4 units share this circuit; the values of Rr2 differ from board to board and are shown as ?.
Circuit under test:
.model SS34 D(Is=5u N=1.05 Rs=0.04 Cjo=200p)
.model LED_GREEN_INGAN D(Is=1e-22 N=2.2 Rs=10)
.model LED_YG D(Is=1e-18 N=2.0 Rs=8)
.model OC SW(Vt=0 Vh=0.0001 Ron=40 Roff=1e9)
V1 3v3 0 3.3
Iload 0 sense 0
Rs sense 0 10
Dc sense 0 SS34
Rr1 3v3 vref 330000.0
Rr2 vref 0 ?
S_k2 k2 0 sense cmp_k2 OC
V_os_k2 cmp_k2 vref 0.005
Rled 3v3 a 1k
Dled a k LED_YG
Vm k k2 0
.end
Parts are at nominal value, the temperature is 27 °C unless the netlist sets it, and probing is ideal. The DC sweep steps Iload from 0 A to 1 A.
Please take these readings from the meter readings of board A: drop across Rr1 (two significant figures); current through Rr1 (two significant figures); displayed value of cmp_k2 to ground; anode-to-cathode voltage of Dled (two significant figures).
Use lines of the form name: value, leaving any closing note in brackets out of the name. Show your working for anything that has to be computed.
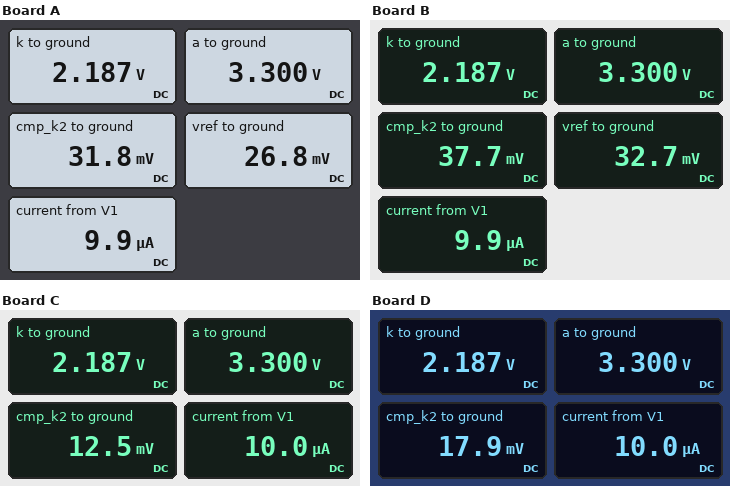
drop across Rr1: 3.3 V - 26.8 mV = 3.3 V
current through Rr1: (3.3 V - 26.8 mV) / 330 kΩ = 9.9 µA
displayed value of cmp_k2 to ground: 31.8 mV
anode-to-cathode voltage of Dled: 3.3 V - 2.187 V = 1.1 V
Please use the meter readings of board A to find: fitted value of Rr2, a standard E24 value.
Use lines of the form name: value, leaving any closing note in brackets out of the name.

fitted value of Rr2, a standard E24 value: 2.7 kΩ
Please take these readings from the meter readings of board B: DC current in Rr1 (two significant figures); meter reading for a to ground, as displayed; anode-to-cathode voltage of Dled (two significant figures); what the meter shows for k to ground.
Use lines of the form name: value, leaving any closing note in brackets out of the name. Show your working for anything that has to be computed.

DC current in Rr1: (3.3 V - 32.7 mV) / 330 kΩ = 9.9 µA
meter reading for a to ground, as displayed: 3.300 V
anode-to-cathode voltage of Dled: 3.3 V - 2.187 V = 1.1 V
what the meter shows for k to ground: 2.187 V
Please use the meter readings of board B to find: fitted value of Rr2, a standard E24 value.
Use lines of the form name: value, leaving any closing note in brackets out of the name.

fitted value of Rr2, a standard E24 value: 3.3 kΩ
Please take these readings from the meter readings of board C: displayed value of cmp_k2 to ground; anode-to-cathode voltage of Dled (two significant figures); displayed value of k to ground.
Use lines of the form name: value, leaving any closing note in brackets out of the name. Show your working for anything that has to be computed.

displayed value of cmp_k2 to ground: 12.5 mV
anode-to-cathode voltage of Dled: 3.3 V - 2.187 V = 1.1 V
displayed value of k to ground: 2.187 V
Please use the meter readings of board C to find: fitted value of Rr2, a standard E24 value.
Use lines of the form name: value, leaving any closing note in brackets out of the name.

fitted value of Rr2, a standard E24 value: 750 Ω
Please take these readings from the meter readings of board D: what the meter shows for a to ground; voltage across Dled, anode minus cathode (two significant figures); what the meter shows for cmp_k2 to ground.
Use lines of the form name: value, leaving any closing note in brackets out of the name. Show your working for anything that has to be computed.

what the meter shows for a to ground: 3.300 V
voltage across Dled, anode minus cathode: 3.3 V - 2.187 V = 1.1 V
what the meter shows for cmp_k2 to ground: 17.9 mV
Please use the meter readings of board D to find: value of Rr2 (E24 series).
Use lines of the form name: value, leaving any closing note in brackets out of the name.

value of Rr2: 1.3 kΩ
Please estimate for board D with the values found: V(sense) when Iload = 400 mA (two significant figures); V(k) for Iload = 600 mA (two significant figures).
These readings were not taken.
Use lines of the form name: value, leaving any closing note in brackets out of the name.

V(sense) when Iload = 400 mA: 320 mV
V(k) for Iload = 600 mA: 57 mV
